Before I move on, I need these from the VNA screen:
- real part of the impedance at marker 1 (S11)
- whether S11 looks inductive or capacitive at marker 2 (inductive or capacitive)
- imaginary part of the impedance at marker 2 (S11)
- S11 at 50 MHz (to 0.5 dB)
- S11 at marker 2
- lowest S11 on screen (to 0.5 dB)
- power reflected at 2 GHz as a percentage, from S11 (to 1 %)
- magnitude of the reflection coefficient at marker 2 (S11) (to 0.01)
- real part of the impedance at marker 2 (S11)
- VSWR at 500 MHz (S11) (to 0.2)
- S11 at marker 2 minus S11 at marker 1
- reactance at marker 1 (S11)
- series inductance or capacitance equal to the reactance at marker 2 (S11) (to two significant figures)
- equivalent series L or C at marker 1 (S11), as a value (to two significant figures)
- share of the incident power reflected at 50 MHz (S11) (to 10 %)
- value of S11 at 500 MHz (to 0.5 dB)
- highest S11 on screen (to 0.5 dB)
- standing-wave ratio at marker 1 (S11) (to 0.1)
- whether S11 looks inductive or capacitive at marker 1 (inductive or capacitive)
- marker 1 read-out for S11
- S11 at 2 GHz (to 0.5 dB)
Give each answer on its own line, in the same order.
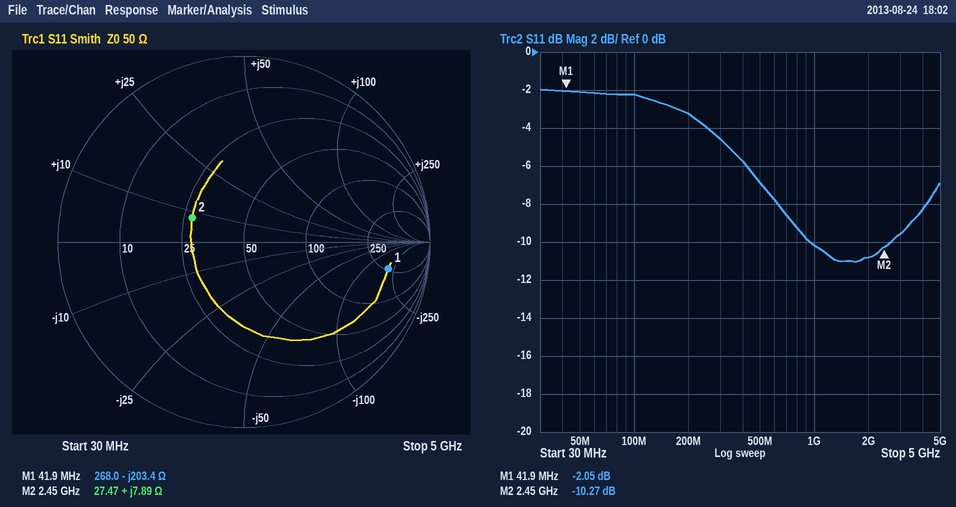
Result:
268.0 Ω
inductive
+7.89 Ω
-2.0 dB
-10.27 dB
-11.0 dB
8 %
0.31
27.47 Ω
2.6
-8.22 dB
-203.4 Ω
510 pH
19 pF
60 %
-7.0 dB
-2.0 dB
8.5
capacitive
-2.05 dB
-11.0 dB
